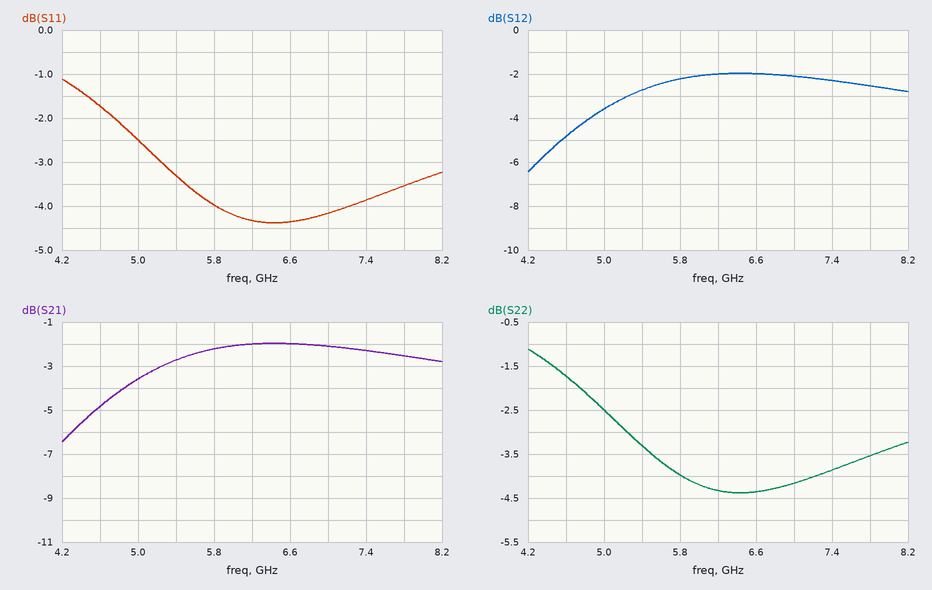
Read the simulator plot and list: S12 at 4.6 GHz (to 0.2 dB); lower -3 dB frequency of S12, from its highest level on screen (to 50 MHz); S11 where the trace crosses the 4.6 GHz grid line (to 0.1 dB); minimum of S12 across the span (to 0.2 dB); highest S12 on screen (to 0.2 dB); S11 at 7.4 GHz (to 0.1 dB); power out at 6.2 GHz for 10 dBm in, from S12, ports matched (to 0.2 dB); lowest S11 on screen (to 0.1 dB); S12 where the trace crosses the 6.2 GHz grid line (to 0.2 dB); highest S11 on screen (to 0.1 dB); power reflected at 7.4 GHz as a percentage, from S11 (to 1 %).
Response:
-4.8 dB
4.55 GHz
-1.7 dB
-6.4 dB
-2.0 dB
-3.9 dB
8.0 dBm
-4.4 dB
-2.0 dB
-1.1 dB
41 %
